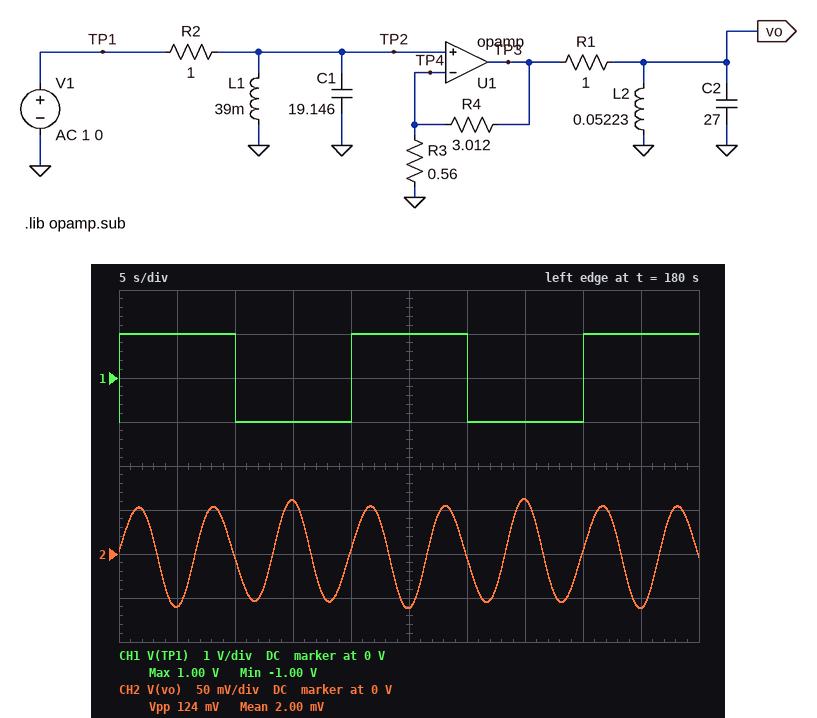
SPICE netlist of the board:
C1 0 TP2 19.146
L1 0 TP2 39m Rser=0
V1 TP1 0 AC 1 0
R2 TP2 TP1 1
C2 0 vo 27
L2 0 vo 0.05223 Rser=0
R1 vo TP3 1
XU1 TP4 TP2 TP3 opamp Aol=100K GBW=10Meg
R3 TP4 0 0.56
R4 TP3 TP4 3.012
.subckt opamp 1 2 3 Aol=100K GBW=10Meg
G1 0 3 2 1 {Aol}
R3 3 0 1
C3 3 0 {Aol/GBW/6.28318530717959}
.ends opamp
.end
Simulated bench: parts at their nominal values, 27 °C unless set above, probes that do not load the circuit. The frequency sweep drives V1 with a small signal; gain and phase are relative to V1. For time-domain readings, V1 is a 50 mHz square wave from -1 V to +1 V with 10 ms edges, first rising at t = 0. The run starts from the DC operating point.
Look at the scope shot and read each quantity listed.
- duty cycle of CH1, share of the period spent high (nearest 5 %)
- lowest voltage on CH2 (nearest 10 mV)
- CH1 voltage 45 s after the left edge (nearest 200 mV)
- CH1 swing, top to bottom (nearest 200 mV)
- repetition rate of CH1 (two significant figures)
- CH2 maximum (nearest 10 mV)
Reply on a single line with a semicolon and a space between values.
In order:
50 %; -60 mV; 1.0 V; 2.0 V; 50 mHz; 60 mV
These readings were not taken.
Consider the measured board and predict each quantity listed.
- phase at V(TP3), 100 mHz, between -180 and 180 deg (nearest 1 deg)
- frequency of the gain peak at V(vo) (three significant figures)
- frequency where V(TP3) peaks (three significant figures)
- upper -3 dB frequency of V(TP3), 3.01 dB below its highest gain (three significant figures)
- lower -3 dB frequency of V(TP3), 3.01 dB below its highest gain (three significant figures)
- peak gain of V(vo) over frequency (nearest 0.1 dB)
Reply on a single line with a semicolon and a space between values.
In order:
88 deg; 134 mHz; 184 mHz; 188 mHz; 180 mHz; -7.0 dB
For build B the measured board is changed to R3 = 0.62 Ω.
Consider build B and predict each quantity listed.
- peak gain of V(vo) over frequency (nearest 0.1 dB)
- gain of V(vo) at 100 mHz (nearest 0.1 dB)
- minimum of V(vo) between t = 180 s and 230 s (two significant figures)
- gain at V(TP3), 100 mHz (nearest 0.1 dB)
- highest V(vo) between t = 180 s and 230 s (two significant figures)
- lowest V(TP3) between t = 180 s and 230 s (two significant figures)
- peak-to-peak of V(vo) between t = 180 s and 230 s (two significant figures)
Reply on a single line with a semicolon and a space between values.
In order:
-7.8 dB; -36.5 dB; -57 mV; -13.8 dB; 57 mV; -330 mV; 110 mV
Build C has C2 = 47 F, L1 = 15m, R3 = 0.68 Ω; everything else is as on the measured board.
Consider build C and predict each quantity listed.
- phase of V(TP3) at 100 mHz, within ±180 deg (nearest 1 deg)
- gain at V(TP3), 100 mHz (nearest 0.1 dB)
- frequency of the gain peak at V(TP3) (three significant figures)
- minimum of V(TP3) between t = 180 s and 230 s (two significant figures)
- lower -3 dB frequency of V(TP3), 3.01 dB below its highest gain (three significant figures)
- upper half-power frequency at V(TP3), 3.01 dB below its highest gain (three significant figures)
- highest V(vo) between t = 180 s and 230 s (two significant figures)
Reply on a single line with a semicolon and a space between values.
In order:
89 deg; -24.8 dB; 297 mHz; -170 mV; 293 mHz; 301 mHz; 3.1 mV
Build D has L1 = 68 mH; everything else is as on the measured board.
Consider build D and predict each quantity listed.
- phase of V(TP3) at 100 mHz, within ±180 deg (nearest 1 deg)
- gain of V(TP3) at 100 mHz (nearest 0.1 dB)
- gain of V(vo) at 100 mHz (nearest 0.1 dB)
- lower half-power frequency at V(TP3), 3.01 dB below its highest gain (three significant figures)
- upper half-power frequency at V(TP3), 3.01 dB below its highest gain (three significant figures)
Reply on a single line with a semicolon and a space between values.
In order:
85 deg; -5.1 dB; -27.7 dB; 135 mHz; 144 mHz
